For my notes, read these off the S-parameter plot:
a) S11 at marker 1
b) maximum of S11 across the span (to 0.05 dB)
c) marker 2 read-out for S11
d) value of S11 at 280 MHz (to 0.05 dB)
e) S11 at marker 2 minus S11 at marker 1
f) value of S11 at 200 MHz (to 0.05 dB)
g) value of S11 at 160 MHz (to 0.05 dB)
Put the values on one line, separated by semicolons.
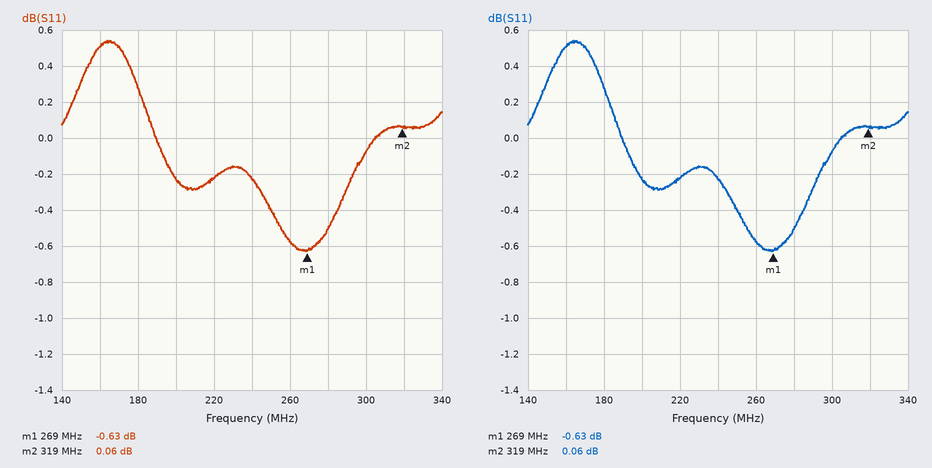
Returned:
-0.63 dB; 0.55 dB; 0.06 dB; -0.50 dB; 0.69 dB; -0.25 dB; 0.50 dB
